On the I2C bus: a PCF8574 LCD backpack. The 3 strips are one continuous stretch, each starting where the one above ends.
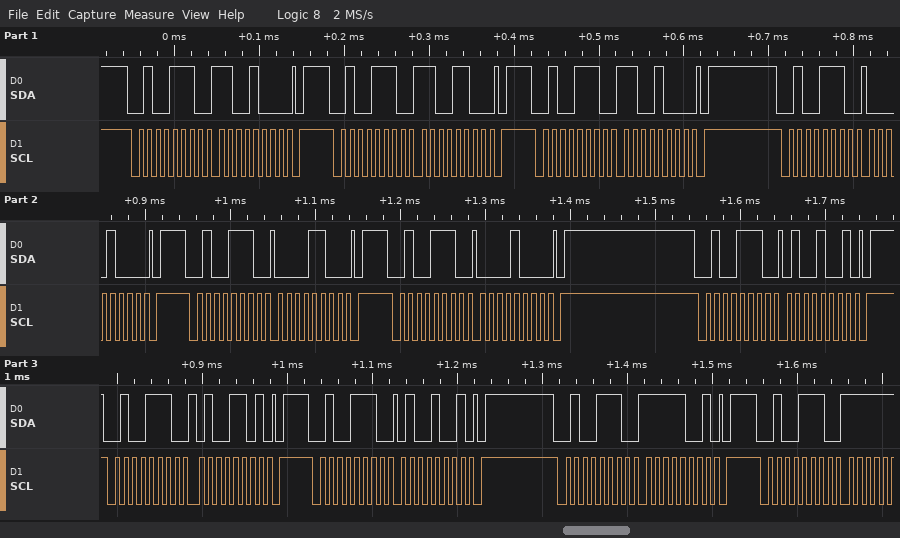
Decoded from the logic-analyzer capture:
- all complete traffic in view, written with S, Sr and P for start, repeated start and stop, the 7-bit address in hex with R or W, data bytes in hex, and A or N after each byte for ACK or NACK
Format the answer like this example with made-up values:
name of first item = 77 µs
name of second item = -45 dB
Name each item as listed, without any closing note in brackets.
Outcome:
all complete traffic in view, written with S, Sr and P for start, repeated start and stop, the 7-bit address in hex with R or W, data bytes in hex, and A or N after each byte for ACK or NACK = S 27W A C8 A P S 27W A CC A P S 27W A C8 A P S 27W A 08 A P S 27W A 0C A P S 27W A 08 A P S 27W A 49 A P S 27W A 4D A P S 27W A 49 A P S 27W A F9 A P S 27W A
